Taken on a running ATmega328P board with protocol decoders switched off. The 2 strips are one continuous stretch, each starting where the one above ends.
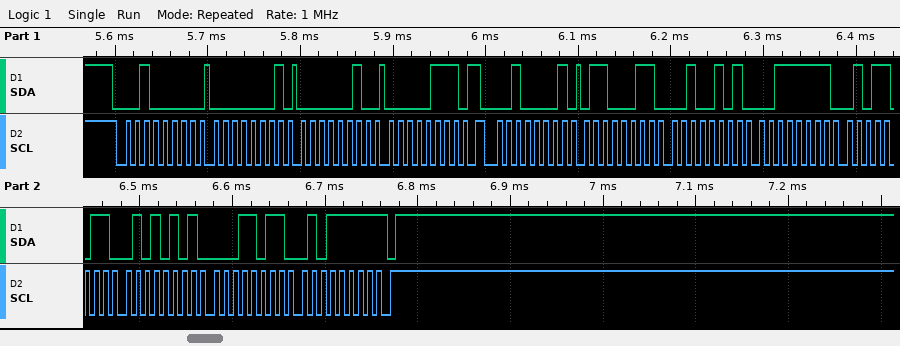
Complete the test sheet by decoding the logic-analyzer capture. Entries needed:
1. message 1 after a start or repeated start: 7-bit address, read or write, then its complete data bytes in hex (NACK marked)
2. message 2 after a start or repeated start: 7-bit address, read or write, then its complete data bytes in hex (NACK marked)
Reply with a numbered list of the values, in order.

1. 0x10 write: 01 02 07
2. 0x10 read: 63 25 3F 5B 55 1B 5F NACK
